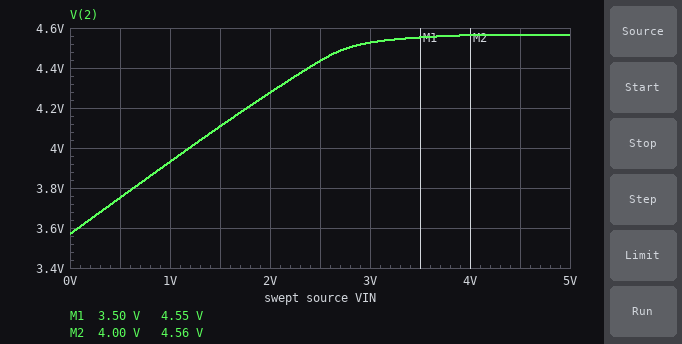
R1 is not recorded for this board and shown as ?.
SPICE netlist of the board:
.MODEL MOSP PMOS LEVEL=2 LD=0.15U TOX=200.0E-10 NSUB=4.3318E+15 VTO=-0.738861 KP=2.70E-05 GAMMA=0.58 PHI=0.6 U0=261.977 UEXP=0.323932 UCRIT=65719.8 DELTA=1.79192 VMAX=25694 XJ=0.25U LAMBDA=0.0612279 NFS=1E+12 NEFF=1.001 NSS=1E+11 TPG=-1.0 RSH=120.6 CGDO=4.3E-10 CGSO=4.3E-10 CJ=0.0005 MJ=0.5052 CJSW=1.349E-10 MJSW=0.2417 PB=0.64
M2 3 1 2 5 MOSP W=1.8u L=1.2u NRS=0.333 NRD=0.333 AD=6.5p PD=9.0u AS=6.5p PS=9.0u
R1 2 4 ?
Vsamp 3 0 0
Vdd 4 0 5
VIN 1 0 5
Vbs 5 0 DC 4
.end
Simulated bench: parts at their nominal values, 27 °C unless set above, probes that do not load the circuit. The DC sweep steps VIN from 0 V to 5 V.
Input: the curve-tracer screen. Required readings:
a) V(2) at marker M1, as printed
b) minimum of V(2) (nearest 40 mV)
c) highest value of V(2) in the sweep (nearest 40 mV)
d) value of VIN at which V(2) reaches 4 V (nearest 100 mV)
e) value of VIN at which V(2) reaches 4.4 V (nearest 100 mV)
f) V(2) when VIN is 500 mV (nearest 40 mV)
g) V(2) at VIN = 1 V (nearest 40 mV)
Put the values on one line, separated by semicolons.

4.55 V; 3.56 V; 4.56 V; 1.2 V; 2.4 V; 3.76 V; 3.92 V
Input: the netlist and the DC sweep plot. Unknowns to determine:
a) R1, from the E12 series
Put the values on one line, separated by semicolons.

15 kΩ
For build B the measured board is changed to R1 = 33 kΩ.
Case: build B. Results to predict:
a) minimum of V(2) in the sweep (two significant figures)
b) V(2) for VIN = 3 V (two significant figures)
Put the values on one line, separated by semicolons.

2.9 V; 4.4 V
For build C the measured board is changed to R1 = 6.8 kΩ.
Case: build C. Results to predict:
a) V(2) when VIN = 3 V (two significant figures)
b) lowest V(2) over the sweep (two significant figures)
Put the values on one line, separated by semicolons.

4.6 V; 4.1 V
